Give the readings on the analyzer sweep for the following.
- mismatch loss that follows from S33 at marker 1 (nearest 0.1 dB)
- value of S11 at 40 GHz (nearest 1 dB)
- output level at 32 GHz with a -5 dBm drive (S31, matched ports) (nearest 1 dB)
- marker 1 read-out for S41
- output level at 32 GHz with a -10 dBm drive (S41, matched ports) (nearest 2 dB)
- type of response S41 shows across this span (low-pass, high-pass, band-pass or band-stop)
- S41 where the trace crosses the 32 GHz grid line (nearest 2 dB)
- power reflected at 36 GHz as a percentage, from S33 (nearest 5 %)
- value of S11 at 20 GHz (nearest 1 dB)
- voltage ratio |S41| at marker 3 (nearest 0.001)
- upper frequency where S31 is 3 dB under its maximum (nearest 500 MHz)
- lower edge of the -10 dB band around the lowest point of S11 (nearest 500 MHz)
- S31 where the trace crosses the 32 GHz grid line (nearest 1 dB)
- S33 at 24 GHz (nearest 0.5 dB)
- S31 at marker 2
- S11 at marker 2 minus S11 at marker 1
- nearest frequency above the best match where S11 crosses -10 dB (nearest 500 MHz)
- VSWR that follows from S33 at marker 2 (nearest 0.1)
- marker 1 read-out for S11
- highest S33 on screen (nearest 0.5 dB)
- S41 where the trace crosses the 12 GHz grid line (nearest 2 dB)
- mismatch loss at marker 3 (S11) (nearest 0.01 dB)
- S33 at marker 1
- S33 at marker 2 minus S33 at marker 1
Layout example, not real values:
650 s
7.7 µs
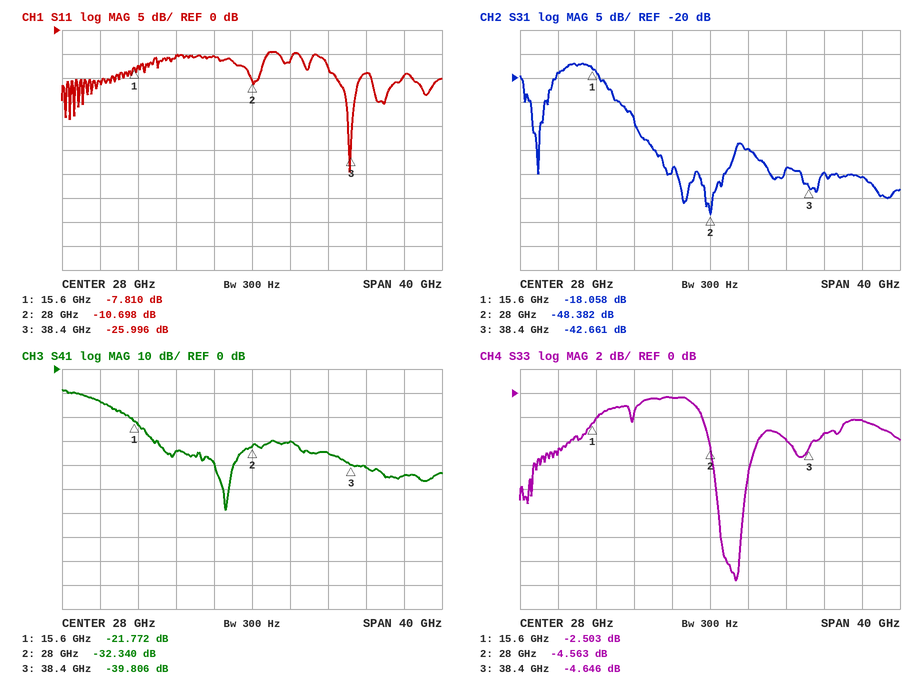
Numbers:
3.6 dB
-9 dB
-40 dBm
-21.772 dB
-40 dBm
low-pass
-30 dB
40 %
-5 dB
0.010
16.5 GHz
37.0 GHz
-35 dB
-0.5 dB
-48.382 dB
-2.888 dB
39.5 GHz
3.9
-7.810 dB
-0.5 dB
-14 dB
0.01 dB
-2.503 dB
-2.060 dB
